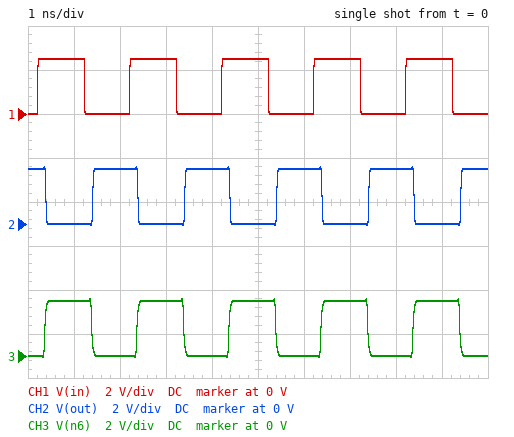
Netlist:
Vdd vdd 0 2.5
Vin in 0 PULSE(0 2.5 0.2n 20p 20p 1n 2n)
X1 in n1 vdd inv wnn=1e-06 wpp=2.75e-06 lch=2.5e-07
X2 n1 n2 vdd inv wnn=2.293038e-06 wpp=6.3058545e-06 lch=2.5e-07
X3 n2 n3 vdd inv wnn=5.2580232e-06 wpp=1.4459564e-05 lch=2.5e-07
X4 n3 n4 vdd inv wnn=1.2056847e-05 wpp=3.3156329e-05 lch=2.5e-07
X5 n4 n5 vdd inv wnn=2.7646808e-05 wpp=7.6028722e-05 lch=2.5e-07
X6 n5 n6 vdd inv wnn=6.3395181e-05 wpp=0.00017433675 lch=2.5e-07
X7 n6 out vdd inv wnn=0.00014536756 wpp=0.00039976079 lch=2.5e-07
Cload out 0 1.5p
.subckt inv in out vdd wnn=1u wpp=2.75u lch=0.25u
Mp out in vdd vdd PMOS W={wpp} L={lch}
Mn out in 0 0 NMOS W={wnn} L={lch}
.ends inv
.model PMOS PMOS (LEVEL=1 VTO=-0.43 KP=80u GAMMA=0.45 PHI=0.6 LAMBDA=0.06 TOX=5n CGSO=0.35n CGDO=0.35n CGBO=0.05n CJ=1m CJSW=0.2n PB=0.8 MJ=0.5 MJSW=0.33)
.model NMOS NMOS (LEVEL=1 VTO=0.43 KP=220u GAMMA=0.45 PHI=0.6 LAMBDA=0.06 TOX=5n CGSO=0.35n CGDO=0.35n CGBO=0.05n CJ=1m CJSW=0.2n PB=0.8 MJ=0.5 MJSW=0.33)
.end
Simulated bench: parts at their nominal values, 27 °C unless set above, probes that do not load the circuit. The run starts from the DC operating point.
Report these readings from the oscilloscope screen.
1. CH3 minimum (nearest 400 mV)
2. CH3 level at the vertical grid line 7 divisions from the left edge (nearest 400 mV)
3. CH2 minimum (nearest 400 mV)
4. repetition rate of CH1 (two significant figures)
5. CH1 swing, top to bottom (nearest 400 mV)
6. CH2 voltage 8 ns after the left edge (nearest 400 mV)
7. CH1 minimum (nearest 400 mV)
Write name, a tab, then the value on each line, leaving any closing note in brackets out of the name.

CH3 minimum	0 V
CH3 level at the vertical grid line 7 divisions from the left edge	2.4 V
CH2 minimum	0 V
repetition rate of CH1	500 MHz
CH1 swing, top to bottom	2.4 V
CH2 voltage 8 ns after the left edge	2.4 V
CH1 minimum	0 V
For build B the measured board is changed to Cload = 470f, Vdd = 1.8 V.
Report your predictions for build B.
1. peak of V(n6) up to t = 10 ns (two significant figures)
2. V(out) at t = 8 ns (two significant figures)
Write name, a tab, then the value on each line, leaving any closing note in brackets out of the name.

peak of V(n6) up to t = 10 ns	1.9 V
V(out) at t = 8 ns	1.8 V
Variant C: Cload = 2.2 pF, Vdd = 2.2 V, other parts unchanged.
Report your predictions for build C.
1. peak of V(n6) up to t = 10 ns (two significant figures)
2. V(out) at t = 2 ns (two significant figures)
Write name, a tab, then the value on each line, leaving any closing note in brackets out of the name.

peak of V(n6) up to t = 10 ns	2.3 V
V(out) at t = 2 ns	2.2 V
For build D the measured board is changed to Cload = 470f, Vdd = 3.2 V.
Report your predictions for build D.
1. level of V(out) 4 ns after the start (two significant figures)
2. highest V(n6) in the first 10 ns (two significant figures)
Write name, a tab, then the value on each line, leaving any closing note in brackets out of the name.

level of V(out) 4 ns after the start	3.2 V
highest V(n6) in the first 10 ns	3.3 V
